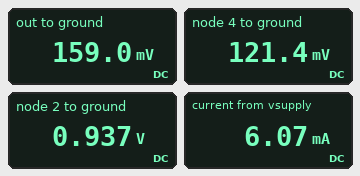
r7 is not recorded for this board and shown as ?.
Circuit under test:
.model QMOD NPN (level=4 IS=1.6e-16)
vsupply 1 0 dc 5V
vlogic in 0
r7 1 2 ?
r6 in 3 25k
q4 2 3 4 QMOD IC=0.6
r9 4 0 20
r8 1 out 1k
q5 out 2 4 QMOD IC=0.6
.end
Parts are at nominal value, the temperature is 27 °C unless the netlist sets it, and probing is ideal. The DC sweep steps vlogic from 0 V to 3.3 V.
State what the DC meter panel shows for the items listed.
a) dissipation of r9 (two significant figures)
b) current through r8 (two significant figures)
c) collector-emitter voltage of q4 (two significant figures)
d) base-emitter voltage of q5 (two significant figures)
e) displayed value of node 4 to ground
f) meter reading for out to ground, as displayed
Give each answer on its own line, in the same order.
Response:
740 µW
4.8 mA
820 mV
820 mV
121.4 mV
159.0 mV
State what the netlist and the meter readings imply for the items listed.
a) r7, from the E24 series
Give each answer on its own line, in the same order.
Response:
3.3 kΩ
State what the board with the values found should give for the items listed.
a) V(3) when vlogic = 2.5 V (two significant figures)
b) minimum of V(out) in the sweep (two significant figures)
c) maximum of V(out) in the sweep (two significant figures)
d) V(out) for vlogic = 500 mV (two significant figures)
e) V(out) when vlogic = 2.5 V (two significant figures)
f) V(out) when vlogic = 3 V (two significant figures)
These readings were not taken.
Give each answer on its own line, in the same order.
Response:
810 mV
160 mV
5.0 V
160 mV
5.0 V
5.0 V
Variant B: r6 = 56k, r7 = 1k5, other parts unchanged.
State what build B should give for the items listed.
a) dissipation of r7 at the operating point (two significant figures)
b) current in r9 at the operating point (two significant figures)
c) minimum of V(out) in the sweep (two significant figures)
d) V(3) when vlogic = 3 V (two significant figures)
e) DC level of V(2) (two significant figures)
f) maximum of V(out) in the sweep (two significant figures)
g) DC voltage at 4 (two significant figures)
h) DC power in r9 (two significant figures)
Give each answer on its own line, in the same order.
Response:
11 mW
7.5 mA
180 mV
860 mV
980 mV
5.0 V
150 mV
1.1 mW
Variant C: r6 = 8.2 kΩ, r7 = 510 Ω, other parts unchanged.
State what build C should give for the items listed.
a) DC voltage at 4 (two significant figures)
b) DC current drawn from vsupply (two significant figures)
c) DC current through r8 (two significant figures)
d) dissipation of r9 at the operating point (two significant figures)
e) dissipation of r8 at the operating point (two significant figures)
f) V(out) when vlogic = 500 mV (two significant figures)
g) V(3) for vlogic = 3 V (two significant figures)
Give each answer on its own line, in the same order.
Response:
250 mV
12 mA
4.7 mA
3.1 mW
22 mW
270 mV
1.0 V
